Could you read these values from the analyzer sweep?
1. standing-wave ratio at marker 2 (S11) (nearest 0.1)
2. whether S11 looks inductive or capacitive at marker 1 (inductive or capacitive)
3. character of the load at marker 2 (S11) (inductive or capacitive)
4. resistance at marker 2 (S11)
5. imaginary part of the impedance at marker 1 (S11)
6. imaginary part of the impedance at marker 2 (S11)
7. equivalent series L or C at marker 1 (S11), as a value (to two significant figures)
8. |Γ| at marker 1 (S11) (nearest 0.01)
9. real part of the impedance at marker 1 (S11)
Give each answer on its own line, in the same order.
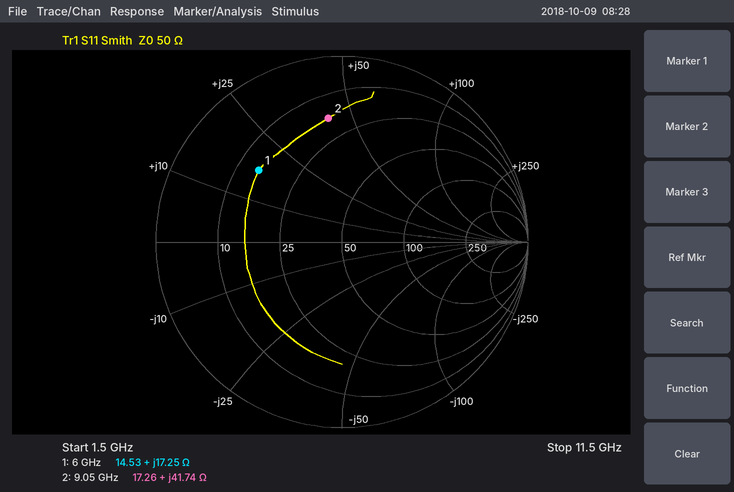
5.1
inductive
inductive
17.26 Ω
+17.25 Ω
+41.74 Ω
460 pH
0.59
14.53 Ω
